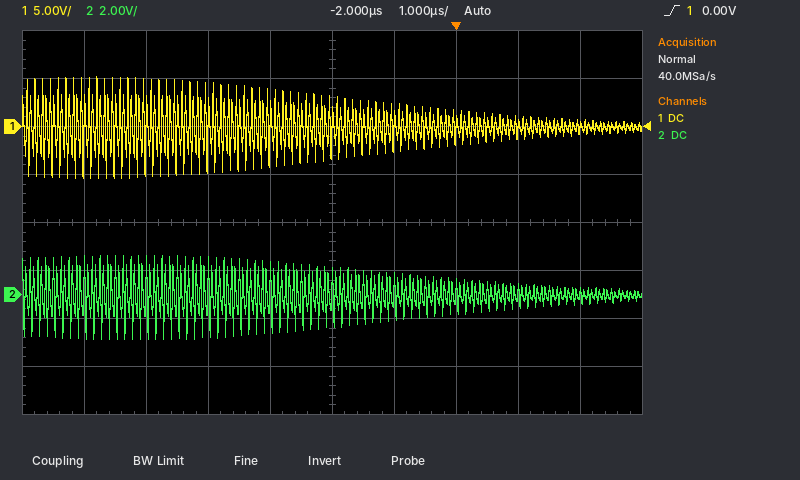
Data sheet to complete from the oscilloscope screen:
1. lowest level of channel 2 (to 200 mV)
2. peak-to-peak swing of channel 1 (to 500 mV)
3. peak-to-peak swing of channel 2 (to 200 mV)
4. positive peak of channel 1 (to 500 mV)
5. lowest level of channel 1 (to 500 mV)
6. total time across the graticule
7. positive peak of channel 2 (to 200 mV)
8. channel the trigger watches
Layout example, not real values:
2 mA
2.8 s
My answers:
-1.8 V
10.5 V
3.4 V
5.0 V
-5.5 V
10 µs
1.6 V
channel 1
